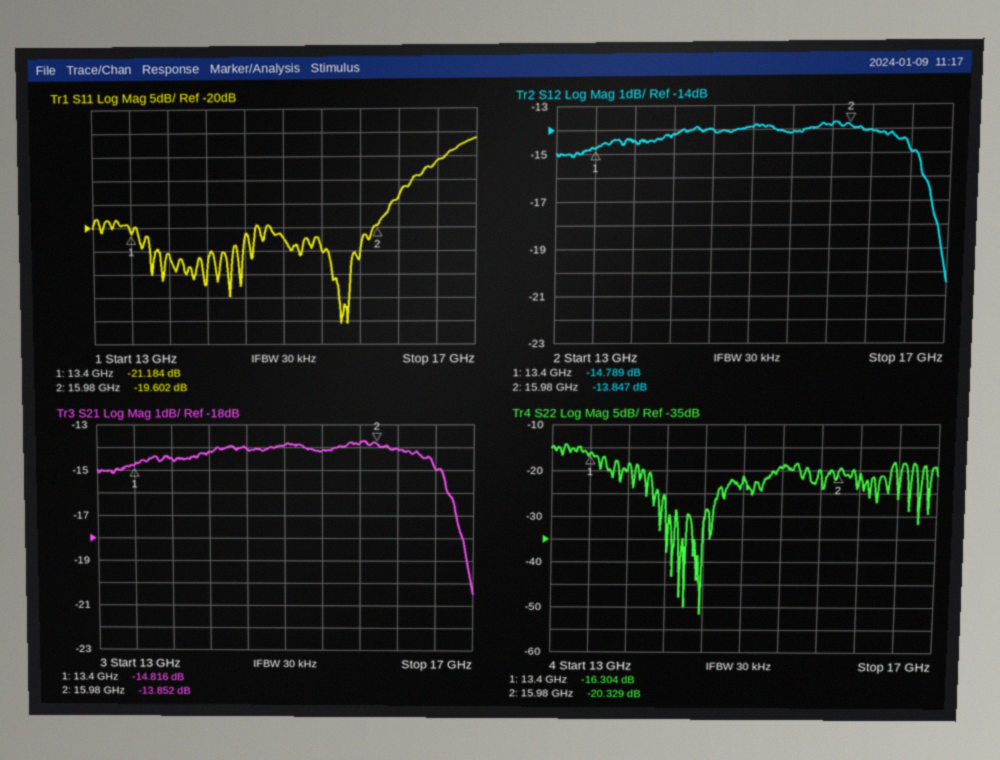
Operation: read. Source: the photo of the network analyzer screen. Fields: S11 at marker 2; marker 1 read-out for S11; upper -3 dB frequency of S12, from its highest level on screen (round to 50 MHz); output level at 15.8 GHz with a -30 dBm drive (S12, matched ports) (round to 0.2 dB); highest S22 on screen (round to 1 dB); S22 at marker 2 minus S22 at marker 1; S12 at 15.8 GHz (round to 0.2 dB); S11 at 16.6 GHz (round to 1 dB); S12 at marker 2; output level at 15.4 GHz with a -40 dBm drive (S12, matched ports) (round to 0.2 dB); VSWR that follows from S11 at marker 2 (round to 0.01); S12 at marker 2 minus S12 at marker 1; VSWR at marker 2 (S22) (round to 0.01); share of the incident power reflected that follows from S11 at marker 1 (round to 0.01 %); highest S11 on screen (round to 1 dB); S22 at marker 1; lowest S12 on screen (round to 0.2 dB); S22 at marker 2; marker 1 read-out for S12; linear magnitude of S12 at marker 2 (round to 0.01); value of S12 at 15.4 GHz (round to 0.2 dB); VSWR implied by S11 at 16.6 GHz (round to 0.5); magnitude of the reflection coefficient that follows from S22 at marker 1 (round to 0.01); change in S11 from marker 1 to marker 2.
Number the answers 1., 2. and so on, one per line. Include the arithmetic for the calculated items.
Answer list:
1. -19.602 dB
2. -21.184 dB
3. 16.80 GHz
4. -30 dBm + (-13.8 dB) = -43.8 dBm
5. -14 dB
6. -20.329 − (-16.304) = -4.025 dB
7. -13.8 dB
8. -6 dB
9. -13.847 dB
10. -40 dBm + (-14.2 dB) = -54.2 dBm
11. (1 + 0.1047)/(1 − 0.1047) ≈ 1.23
12. -13.847 − (-14.789) = 0.942 dB
13. (1 + 0.0963)/(1 − 0.0963) ≈ 1.21
14. 10^(-21.184/10) ≈ 0.76 %
15. -1 dB
16. -16.304 dB
17. -20.4 dB
18. -20.329 dB
19. -14.789 dB
20. 10^(-13.847/20) ≈ 0.20
21. -14.2 dB
22. |Γ| = 10^(-6/20) = 0.5012; VSWR = (1 + 0.5012)/(1 − 0.5012) ≈ 3.0
23. 10^(-16.304/20) ≈ 0.15
24. -19.602 − (-21.184) = 1.582 dB
